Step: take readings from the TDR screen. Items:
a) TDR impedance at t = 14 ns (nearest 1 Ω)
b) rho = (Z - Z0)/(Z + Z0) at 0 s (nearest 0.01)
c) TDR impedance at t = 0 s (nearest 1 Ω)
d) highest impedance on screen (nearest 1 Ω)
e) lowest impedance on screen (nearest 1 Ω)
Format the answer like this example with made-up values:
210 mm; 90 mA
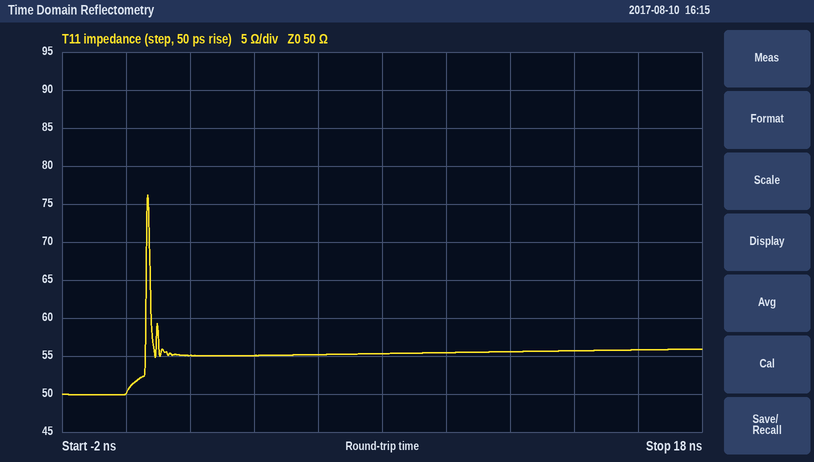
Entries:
56 Ω; 0.00; 50 Ω; 76 Ω; 50 Ω
